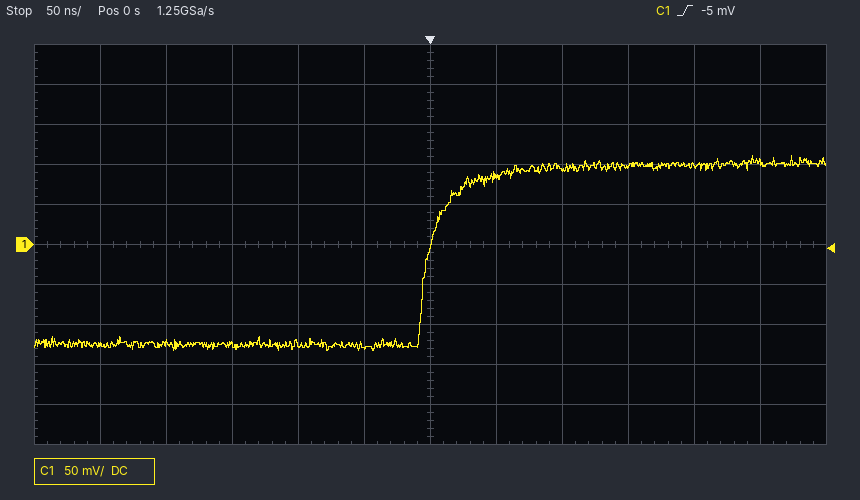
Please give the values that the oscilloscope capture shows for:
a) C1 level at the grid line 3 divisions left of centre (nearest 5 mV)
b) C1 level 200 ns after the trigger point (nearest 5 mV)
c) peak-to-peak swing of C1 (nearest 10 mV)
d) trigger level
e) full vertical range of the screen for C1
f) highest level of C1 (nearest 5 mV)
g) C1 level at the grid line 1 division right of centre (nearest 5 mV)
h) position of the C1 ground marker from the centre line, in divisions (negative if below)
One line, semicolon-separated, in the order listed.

-125 mV; 100 mV; 240 mV; -5 mV; 500 mV; 110 mV; 85 mV; 0.0 div
